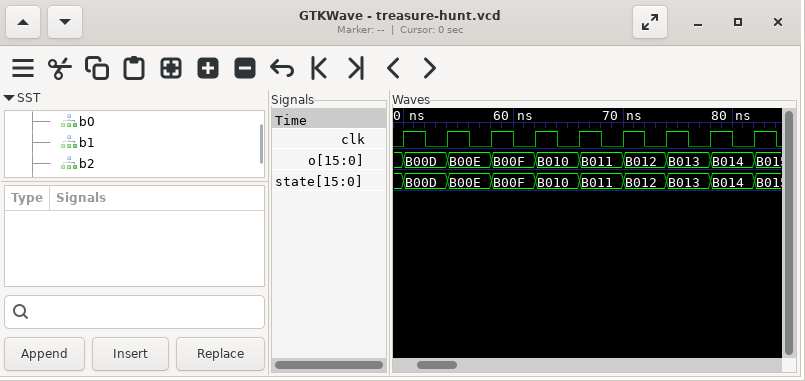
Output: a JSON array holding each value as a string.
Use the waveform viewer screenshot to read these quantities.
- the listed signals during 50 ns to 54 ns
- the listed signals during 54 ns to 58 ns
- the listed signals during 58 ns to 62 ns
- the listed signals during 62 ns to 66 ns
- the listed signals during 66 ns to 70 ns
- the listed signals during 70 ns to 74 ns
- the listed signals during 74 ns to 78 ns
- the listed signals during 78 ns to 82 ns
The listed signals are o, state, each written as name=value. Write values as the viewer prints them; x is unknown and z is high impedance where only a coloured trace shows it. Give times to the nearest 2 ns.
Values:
["o=B00D, state=B00D", "o=B00E, state=B00E", "o=B00F, state=B00F", "o=B010, state=B010", "o=B011, state=B011", "o=B012, state=B012", "o=B013, state=B013", "o=B014, state=B014"]
